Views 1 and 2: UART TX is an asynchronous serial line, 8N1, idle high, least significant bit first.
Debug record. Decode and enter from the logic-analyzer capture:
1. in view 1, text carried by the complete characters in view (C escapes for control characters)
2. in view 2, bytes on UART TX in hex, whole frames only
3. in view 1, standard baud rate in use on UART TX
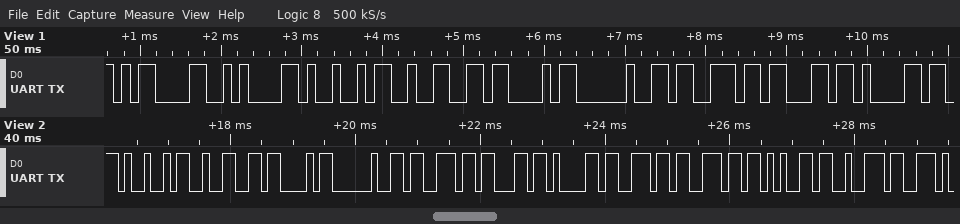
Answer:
"\r\nI2C sca"
49 32 43 20 73 63 61 6E 6E 65 72
9600 baud
